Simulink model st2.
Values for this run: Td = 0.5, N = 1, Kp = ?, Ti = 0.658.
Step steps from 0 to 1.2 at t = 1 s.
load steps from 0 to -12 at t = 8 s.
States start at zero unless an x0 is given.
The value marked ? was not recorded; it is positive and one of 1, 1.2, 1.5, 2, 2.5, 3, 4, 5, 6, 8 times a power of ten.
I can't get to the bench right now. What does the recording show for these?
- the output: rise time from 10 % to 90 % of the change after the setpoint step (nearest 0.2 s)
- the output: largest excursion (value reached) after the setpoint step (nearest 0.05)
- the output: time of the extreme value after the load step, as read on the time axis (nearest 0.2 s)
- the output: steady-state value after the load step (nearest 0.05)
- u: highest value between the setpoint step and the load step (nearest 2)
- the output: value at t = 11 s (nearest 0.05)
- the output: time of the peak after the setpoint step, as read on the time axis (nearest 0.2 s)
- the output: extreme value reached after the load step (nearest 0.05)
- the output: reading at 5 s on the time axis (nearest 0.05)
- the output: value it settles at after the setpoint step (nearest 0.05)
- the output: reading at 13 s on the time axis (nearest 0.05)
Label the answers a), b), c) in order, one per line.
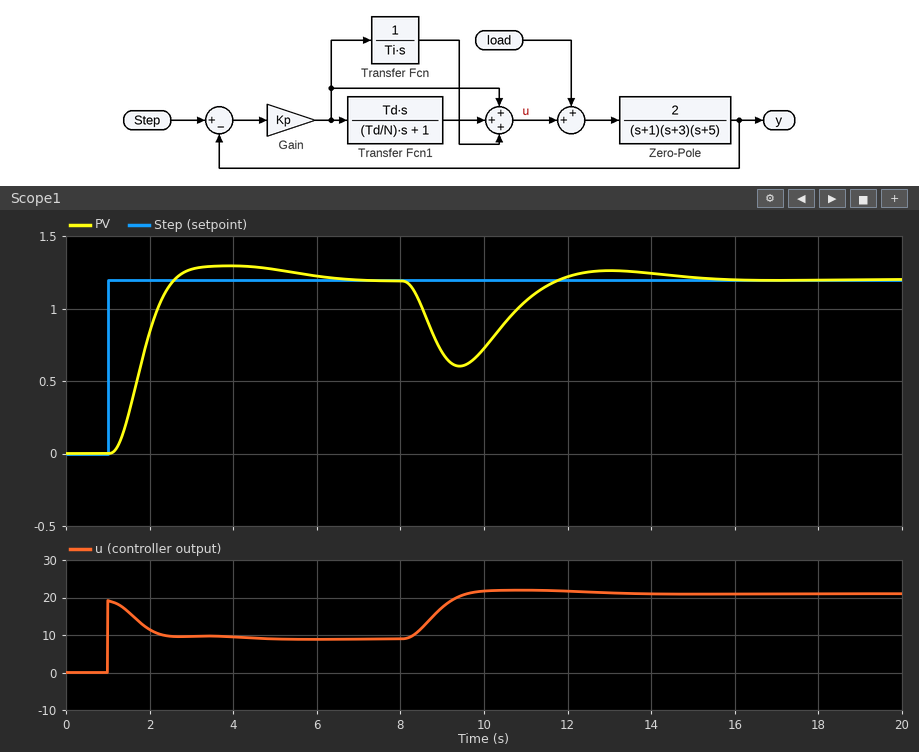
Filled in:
a) 1.0 s
b) 1.30
c) 9.4 s
d) 1.20
e) 20
f) 1.05
g) 4.0 s
h) 0.60
i) 1.25
j) 1.20
k) 1.25
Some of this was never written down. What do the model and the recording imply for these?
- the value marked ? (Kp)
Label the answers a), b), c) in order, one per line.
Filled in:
a) 8
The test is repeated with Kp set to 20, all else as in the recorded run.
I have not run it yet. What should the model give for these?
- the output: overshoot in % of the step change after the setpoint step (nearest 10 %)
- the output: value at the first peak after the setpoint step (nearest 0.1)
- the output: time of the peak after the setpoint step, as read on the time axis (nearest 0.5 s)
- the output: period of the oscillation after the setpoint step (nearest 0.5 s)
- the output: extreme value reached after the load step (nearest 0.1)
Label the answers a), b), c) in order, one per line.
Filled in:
a) 40 %
b) 1.6
c) 2.0 s
d) 2.0 s
e) 0.8
